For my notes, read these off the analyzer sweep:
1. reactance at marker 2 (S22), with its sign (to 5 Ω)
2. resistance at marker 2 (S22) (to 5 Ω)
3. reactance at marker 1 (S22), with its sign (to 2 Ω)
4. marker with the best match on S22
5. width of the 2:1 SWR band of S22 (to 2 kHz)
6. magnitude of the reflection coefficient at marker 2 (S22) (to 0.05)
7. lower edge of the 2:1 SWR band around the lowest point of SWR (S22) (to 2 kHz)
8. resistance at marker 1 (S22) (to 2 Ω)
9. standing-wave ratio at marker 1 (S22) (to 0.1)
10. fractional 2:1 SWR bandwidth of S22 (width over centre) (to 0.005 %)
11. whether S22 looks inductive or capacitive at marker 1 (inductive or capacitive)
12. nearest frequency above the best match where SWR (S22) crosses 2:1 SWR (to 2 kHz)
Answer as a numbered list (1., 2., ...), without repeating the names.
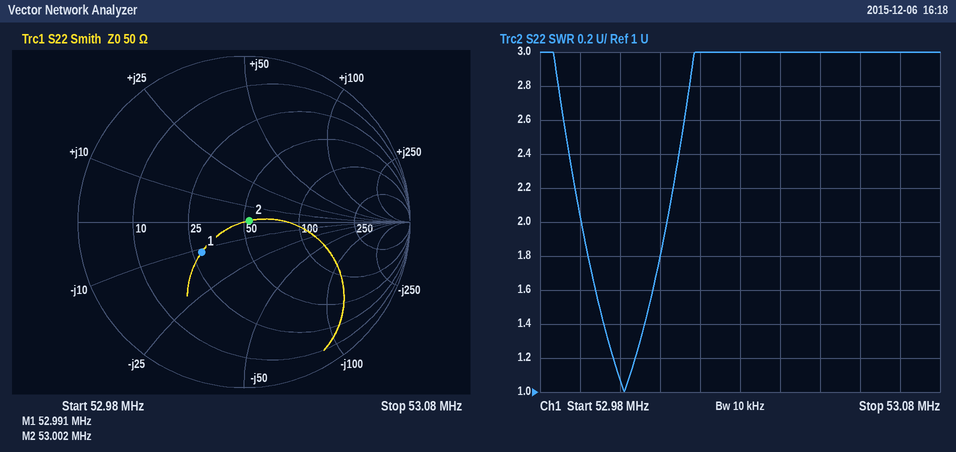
1. 0 Ω
2. 55 Ω
3. -12 Ω
4. marker 2
5. 22 kHz
6. 0.05
7. 52.990 MHz
8. 28 Ω
9. 1.9
10. 0.040 %
11. capacitive
12. 53.012 MHz
